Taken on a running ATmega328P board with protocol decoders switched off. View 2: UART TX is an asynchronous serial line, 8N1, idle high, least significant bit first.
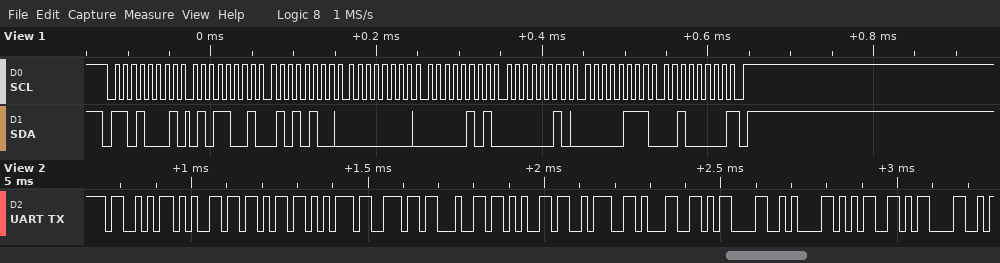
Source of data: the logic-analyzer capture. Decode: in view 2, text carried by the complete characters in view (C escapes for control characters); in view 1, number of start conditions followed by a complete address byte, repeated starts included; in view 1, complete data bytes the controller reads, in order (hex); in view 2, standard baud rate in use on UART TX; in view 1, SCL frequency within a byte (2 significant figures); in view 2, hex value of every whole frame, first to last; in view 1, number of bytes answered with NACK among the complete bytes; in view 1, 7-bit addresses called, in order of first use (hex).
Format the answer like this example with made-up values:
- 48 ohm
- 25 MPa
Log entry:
- "Sekunde:1\r\n5\r"
- 1
- 59 54 00 05 02 07 20
- 57600 baud
- 100 kHz
- 0x53 0x65 0x6B 0x75 0x6E 0x64 0x65 0x3A 0x31 0x0D 0x0A 0x35 0x0D
- 1
- 0x68
